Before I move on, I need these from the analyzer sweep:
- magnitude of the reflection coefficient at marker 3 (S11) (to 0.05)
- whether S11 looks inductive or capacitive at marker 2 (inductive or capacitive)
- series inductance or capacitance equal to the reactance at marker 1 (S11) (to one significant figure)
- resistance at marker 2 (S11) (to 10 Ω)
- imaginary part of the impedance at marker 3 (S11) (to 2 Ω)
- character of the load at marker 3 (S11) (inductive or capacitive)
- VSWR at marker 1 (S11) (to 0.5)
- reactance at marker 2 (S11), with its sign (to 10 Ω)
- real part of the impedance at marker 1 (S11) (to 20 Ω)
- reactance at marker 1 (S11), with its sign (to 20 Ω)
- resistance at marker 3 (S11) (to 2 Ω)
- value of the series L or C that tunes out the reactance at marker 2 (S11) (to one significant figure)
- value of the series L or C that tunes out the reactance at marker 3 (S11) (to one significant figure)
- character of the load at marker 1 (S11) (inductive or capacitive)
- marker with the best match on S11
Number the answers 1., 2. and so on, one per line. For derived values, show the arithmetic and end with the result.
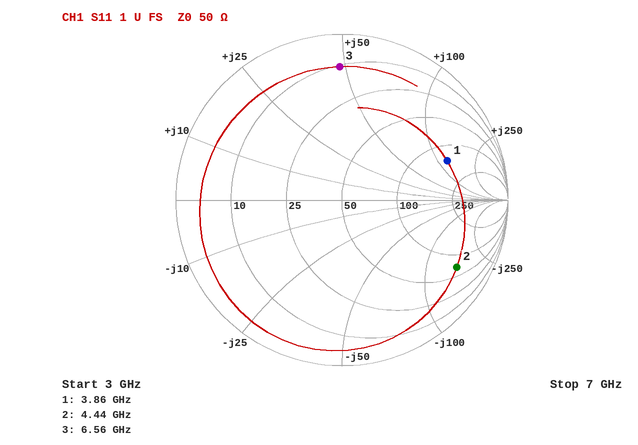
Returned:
1. 0.80
2. capacitive
3. L = 120 Ω/(2π × 3.86 GHz) ≈ 5 nH
4. 70 Ω
5. +48 Ω
6. inductive
7. 5.0
8. -160 Ω
9. 140 Ω
10. +120 Ω
11. 10 Ω
12. L = 160 Ω/(2π × 4.44 GHz) ≈ 6 nH
13. C = 1/(2π × 6.56 GHz × 48 Ω) ≈ 505 fF, so 500 fF to one significant figure
14. inductive
15. marker 1
